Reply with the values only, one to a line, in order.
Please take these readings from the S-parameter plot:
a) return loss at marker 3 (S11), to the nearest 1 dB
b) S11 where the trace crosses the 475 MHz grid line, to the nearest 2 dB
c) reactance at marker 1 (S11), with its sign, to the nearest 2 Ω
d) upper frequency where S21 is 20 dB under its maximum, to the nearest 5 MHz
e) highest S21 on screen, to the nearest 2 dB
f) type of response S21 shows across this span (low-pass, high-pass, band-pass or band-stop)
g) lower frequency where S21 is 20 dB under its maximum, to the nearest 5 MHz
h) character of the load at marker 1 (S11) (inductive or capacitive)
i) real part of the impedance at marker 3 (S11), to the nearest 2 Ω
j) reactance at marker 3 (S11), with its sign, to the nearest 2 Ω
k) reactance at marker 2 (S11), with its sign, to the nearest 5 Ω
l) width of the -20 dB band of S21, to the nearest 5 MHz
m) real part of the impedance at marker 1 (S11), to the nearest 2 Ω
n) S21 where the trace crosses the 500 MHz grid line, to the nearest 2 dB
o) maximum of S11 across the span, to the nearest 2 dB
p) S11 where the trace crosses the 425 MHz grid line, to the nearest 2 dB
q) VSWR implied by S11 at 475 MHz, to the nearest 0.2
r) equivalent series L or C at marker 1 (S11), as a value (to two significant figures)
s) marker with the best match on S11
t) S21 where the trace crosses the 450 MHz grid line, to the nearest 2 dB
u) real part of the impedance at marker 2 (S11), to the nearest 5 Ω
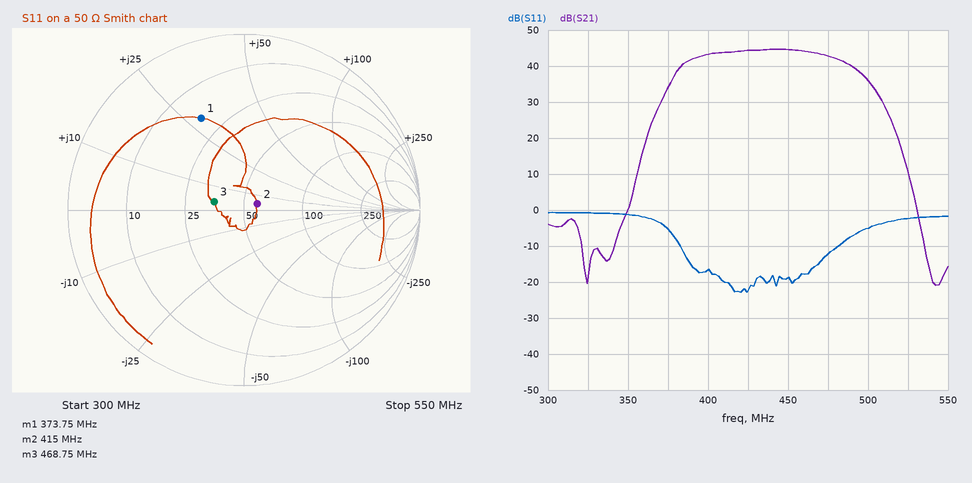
15 dB
-12 dB
+28 Ω
515 MHz
44 dB
band-pass
365 MHz
inductive
36 Ω
+4 Ω
+5 Ω
150 MHz
18 Ω
36 dB
0 dB
-22 dB
1.6
12 nH
marker 2
44 dB
60 Ω
